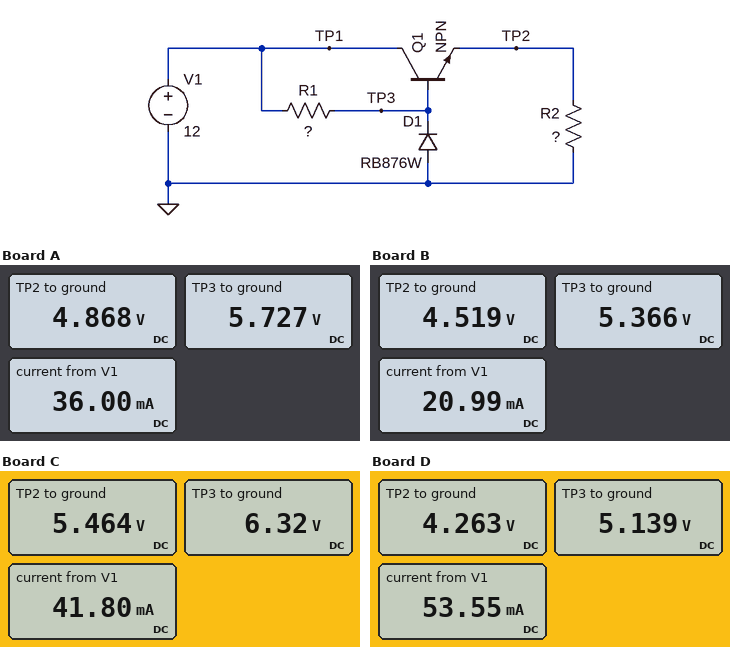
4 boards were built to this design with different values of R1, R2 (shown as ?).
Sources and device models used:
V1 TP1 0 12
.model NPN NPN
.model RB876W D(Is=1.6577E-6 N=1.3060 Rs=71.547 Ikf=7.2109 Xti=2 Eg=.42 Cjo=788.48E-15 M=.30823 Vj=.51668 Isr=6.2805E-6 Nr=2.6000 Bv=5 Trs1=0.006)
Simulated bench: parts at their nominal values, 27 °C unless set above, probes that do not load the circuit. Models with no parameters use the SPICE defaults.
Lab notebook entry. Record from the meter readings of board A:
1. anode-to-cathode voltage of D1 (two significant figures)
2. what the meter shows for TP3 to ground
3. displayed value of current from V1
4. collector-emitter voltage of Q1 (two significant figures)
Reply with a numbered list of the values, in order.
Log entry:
1. -5.7 V
2. 5.727 V
3. 36.00 mA
4. 7.1 V
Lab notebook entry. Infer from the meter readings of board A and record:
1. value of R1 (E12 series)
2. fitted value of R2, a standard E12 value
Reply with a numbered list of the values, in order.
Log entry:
1. 680 Ω
2. 180 Ω
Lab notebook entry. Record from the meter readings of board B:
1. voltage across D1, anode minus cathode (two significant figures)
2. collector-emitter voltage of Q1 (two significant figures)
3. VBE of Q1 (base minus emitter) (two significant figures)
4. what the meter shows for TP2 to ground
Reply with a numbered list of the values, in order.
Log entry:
1. -5.4 V
2. 7.5 V
3. 850 mV
4. 4.519 V
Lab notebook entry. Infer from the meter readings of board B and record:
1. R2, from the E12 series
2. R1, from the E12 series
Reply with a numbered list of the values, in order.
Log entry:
1. 270 Ω
2. 1.5 kΩ
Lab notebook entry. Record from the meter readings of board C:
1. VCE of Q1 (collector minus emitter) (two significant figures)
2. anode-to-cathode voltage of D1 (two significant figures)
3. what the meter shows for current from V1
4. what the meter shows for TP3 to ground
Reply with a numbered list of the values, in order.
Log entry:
1. 6.5 V
2. -6.3 V
3. 41.80 mA
4. 6.32 V
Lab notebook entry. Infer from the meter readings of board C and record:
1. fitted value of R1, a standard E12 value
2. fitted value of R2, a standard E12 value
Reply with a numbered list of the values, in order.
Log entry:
1. 330 Ω
2. 220 Ω
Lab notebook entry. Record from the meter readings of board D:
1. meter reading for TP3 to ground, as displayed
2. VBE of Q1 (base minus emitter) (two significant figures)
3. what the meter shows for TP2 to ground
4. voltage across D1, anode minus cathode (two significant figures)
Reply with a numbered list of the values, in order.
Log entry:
1. 5.139 V
2. 880 mV
3. 4.263 V
4. -5.1 V
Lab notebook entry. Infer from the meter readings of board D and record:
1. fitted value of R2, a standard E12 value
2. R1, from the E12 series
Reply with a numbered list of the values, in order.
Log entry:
1. 82 Ω
2. 3.3 kΩ
